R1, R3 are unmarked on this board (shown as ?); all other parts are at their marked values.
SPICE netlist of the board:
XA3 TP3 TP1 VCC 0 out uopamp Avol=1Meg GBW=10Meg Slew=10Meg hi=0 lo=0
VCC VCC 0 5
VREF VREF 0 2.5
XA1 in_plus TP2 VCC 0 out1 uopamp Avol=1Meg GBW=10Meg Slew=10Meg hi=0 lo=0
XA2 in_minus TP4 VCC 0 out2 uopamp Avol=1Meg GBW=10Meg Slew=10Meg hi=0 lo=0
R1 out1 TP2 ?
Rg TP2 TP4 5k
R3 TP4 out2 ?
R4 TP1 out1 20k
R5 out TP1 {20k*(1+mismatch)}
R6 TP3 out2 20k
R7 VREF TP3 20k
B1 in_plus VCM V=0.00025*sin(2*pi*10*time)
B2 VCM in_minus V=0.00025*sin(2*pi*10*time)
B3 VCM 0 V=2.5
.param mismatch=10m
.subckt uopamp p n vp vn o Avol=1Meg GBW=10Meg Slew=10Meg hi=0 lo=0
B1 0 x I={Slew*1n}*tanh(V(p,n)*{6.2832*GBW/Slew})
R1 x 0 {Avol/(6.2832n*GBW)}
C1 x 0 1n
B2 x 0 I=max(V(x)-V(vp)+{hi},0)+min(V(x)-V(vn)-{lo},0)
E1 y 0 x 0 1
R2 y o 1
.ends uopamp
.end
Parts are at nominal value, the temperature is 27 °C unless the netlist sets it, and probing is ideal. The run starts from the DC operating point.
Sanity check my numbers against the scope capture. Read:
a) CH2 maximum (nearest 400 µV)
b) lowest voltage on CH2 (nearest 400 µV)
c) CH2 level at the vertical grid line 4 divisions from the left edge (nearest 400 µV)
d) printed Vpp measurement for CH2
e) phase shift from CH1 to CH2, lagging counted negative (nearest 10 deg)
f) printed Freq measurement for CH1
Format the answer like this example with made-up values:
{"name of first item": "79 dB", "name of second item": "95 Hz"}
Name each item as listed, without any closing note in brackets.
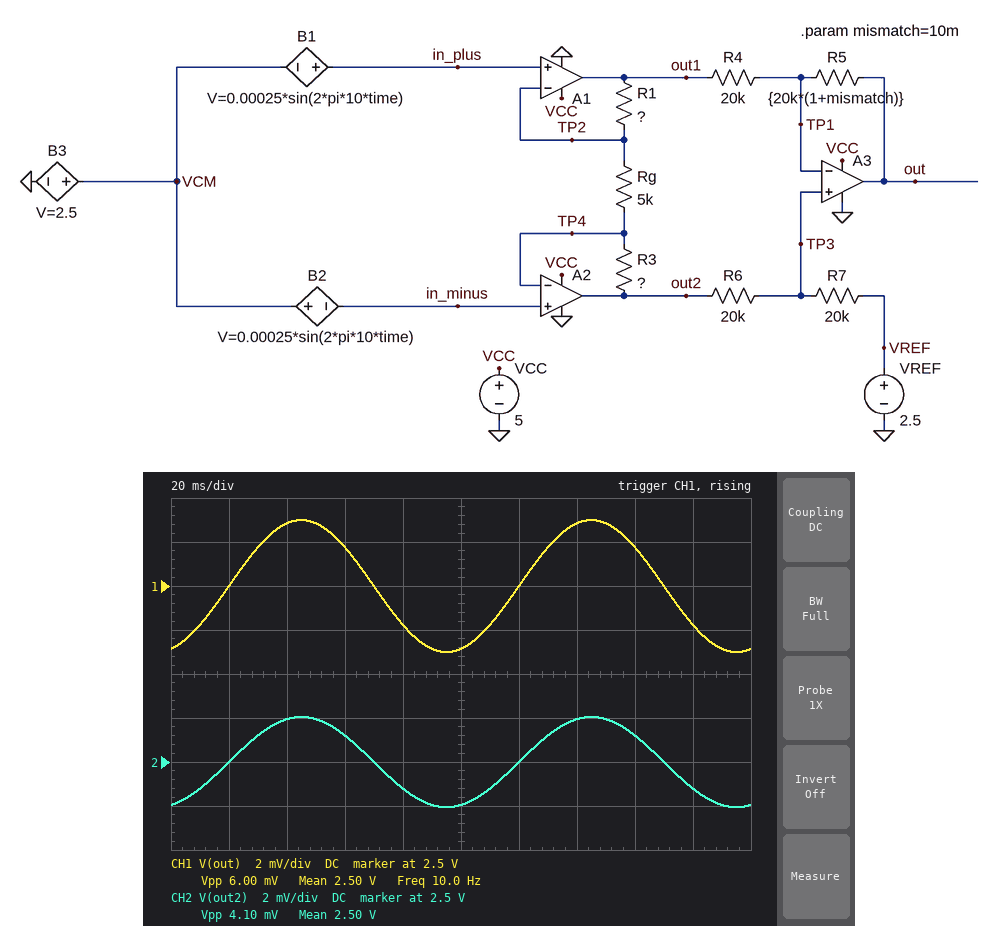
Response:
{"CH2 maximum": "2.5020 V", "lowest voltage on CH2": "2.4980 V", "CH2 level at the vertical grid line 4 divisions from the left edge": "2.4988 V", "printed Vpp measurement for CH2": "4.10 mV", "phase shift from CH1 to CH2, lagging counted negative": "0 deg", "printed Freq measurement for CH1": "10.0 Hz"}
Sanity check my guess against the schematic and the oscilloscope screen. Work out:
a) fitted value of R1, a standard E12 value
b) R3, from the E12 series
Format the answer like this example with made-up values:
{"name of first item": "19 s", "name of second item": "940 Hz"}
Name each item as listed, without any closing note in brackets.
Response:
{"fitted value of R1, a standard E12 value": "6.8 kΩ", "R3, from the E12 series": "18 kΩ"}
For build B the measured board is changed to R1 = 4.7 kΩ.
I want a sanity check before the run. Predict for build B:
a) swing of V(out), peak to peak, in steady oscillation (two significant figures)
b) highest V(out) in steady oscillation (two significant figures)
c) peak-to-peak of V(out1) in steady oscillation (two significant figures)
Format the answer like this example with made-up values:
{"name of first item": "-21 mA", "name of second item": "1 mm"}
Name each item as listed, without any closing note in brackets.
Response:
{"swing of V(out), peak to peak, in steady oscillation": "5.6 mV", "highest V(out) in steady oscillation": "2.5 V", "peak-to-peak of V(out1) in steady oscillation": "1.4 mV"}
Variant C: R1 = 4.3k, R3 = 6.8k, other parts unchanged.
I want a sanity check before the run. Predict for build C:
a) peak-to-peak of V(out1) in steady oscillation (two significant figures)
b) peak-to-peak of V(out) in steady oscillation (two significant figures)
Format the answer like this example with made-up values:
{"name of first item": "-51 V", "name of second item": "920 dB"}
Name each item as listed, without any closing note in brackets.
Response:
{"peak-to-peak of V(out1) in steady oscillation": "1.4 mV", "peak-to-peak of V(out) in steady oscillation": "3.2 mV"}
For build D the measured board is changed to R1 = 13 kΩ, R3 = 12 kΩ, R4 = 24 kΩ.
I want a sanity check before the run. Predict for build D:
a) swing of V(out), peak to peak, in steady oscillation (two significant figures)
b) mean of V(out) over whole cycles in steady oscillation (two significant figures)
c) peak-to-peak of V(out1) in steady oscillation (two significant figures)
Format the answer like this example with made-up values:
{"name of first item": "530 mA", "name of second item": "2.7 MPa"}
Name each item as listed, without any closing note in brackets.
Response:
{"swing of V(out), peak to peak, in steady oscillation": "5.3 mV", "mean of V(out) over whole cycles in steady oscillation": "2.5 V", "peak-to-peak of V(out1) in steady oscillation": "3.1 mV"}
